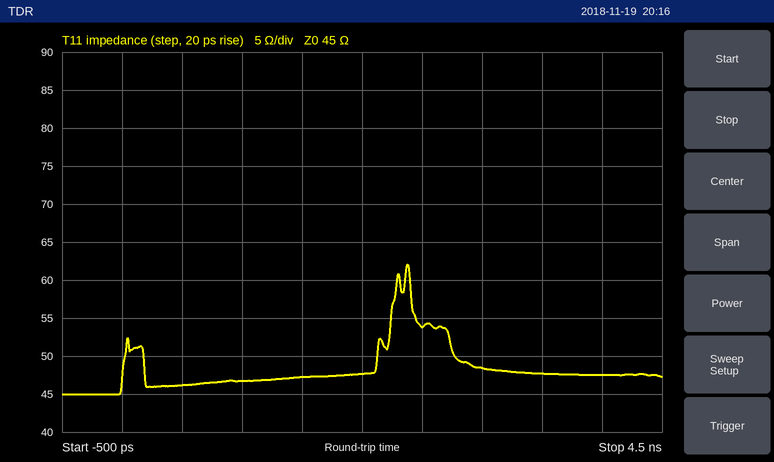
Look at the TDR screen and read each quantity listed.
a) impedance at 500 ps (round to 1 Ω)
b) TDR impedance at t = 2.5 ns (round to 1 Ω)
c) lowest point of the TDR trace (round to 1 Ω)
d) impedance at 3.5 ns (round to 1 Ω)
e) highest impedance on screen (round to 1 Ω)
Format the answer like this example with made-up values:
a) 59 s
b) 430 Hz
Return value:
a) 46 Ω
b) 54 Ω
c) 45 Ω
d) 48 Ω
e) 62 Ω
